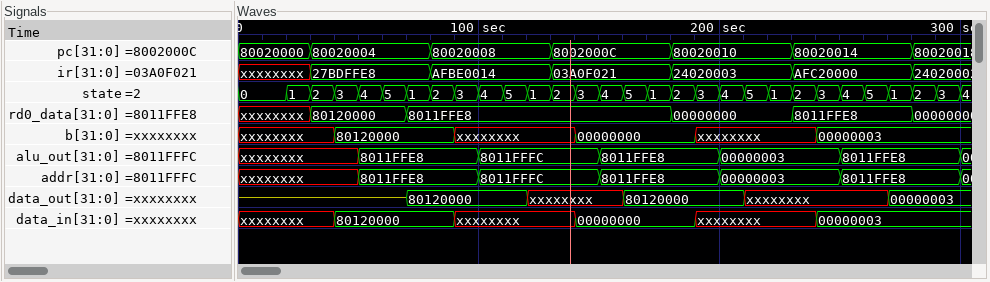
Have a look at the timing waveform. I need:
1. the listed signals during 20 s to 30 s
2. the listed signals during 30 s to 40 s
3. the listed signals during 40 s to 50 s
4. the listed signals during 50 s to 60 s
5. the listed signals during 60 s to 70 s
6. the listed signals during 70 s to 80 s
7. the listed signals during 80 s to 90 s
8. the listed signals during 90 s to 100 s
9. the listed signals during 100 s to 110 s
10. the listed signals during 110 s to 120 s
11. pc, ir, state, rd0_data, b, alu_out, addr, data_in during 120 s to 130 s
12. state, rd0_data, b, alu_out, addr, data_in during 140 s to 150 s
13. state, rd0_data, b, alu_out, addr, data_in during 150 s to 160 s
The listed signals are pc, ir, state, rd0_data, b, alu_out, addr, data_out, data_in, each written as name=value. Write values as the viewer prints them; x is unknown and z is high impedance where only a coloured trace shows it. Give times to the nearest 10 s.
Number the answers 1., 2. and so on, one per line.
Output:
1. pc=80020000, ir=xxxxxxxx, state=1, rd0_data=xxxxxxxx, b=xxxxxxxx, alu_out=xxxxxxxx, addr=xxxxxxxx, data_out=z, data_in=xxxxxxxx
2. pc=80020004, ir=27BDFFE8, state=2, rd0_data=80120000, b=xxxxxxxx, alu_out=xxxxxxxx, addr=xxxxxxxx, data_out=z, data_in=xxxxxxxx
3. pc=80020004, ir=27BDFFE8, state=3, rd0_data=80120000, b=80120000, alu_out=xxxxxxxx, addr=xxxxxxxx, data_out=z, data_in=80120000
4. pc=80020004, ir=27BDFFE8, state=4, rd0_data=80120000, b=80120000, alu_out=8011FFE8, addr=8011FFE8, data_out=z, data_in=80120000
5. pc=80020004, ir=27BDFFE8, state=5, rd0_data=80120000, b=80120000, alu_out=8011FFE8, addr=8011FFE8, data_out=z, data_in=80120000
6. pc=80020004, ir=27BDFFE8, state=1, rd0_data=8011FFE8, b=80120000, alu_out=8011FFE8, addr=8011FFE8, data_out=80120000, data_in=80120000
7. pc=80020008, ir=AFBE0014, state=2, rd0_data=8011FFE8, b=80120000, alu_out=8011FFE8, addr=8011FFE8, data_out=80120000, data_in=80120000
8. pc=80020008, ir=AFBE0014, state=3, rd0_data=8011FFE8, b=xxxxxxxx, alu_out=8011FFE8, addr=8011FFE8, data_out=80120000, data_in=xxxxxxxx
9. pc=80020008, ir=AFBE0014, state=4, rd0_data=8011FFE8, b=xxxxxxxx, alu_out=8011FFFC, addr=8011FFFC, data_out=80120000, data_in=xxxxxxxx
10. pc=80020008, ir=AFBE0014, state=5, rd0_data=8011FFE8, b=xxxxxxxx, alu_out=8011FFFC, addr=8011FFFC, data_out=80120000, data_in=xxxxxxxx
11. pc=80020008, ir=AFBE0014, state=1, rd0_data=8011FFE8, b=xxxxxxxx, alu_out=8011FFFC, addr=8011FFFC, data_in=xxxxxxxx
12. state=3, rd0_data=8011FFE8, b=00000000, alu_out=8011FFFC, addr=8011FFFC, data_in=00000000
13. state=4, rd0_data=8011FFE8, b=00000000, alu_out=8011FFE8, addr=8011FFE8, data_in=00000000
